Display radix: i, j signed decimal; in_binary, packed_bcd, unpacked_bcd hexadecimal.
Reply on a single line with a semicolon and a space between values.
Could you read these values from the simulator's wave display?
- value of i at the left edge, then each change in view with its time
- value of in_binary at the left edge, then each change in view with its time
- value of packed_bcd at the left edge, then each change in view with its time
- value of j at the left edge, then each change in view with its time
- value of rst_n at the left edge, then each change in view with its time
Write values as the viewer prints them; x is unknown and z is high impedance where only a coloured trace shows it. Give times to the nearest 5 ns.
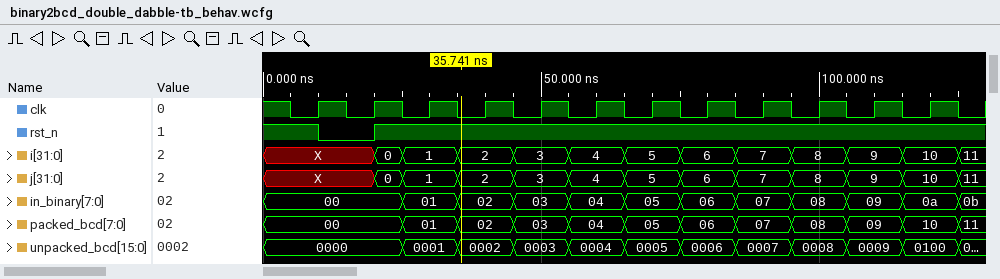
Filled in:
X, 0 at 20 ns, 1 at 25 ns, 2 at 35 ns, 3 at 45 ns, 4 at 55 ns, 5 at 65 ns, 6 at 75 ns, 7 at 85 ns, 8 at 95 ns, 9 at 105 ns, 10 at 115 ns, 11 at 125 ns; 00, 01 at 25 ns, 02 at 35 ns, 03 at 45 ns, 04 at 55 ns, 05 at 65 ns, 06 at 75 ns, 07 at 85 ns, 08 at 95 ns, 09 at 105 ns, 0a at 115 ns, 0b at 125 ns; 00, 01 at 25 ns, 02 at 35 ns, 03 at 45 ns, 04 at 55 ns, 05 at 65 ns, 06 at 75 ns, 07 at 85 ns, 08 at 95 ns, 09 at 105 ns, 10 at 115 ns, 11 at 125 ns; X, 0 at 20 ns, 1 at 25 ns, 2 at 35 ns, 3 at 45 ns, 4 at 55 ns, 5 at 65 ns, 6 at 75 ns, 7 at 85 ns, 8 at 95 ns, 9 at 105 ns, 10 at 115 ns, 11 at 125 ns; 1, 0 at 10 ns, 1 at 20 ns
